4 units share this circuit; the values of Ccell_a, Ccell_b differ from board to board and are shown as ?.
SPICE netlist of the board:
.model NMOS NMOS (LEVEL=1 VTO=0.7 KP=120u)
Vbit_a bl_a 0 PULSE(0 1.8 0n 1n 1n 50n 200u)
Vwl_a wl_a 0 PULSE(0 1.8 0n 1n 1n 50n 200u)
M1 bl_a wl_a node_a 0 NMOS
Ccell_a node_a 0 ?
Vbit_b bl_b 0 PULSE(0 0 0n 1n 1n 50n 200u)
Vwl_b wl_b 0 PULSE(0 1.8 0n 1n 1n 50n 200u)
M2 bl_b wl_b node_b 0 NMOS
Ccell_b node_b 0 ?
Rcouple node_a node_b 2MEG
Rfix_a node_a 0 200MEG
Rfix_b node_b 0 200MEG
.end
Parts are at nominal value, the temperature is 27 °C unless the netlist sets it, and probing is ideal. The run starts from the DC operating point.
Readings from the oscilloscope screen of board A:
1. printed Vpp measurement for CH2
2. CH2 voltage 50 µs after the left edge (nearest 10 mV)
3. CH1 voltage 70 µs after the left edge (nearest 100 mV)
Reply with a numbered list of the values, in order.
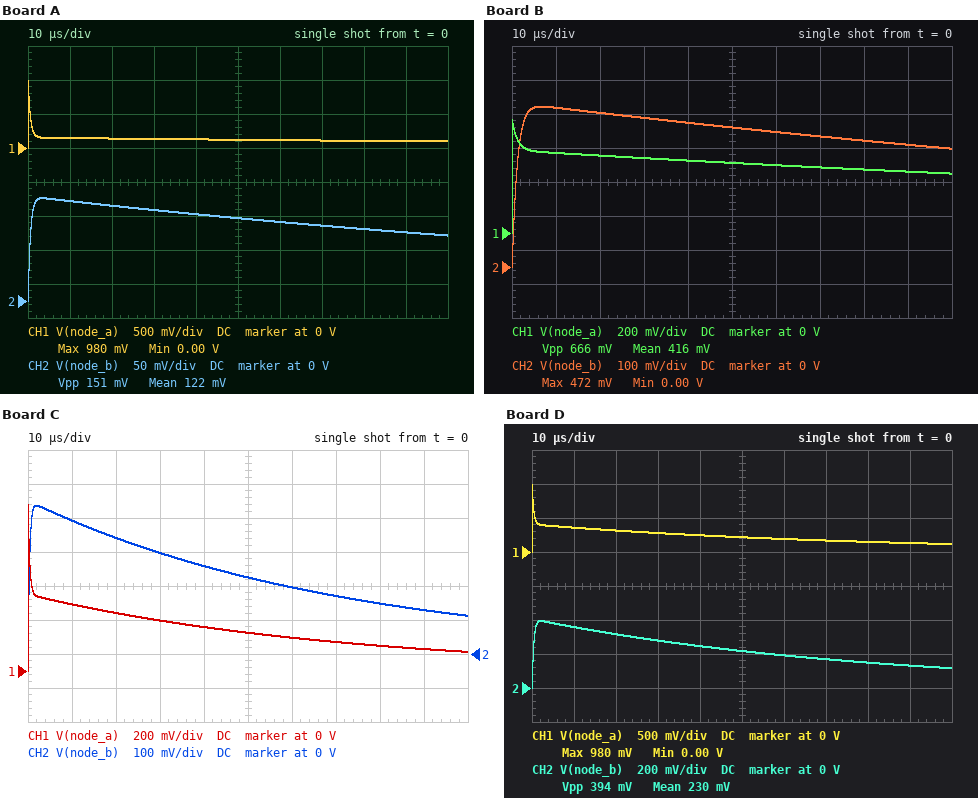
1. 151 mV
2. 120 mV
3. 100 mV
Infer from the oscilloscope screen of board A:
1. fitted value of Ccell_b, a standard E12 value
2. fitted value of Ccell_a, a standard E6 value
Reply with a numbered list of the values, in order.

1. 1.8 pF
2. 330 fF
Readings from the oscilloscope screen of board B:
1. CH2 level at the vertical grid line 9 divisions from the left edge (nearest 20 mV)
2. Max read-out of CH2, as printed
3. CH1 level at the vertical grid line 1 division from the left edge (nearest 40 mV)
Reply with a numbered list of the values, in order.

1. 360 mV
2. 472 mV
3. 480 mV
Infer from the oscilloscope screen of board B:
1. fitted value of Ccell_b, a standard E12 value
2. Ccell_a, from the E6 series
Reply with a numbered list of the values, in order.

1. 820 fF
2. 2.2 pF
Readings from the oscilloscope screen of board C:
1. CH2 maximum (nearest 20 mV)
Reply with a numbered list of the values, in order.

1. 440 mV
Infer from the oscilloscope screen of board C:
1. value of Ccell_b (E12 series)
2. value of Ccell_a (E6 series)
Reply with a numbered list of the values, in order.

1. 390 fF
2. 330 fF
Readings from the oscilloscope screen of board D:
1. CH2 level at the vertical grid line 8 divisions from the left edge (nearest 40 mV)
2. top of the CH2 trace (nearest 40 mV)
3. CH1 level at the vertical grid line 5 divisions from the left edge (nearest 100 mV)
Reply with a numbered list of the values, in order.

1. 160 mV
2. 400 mV
3. 200 mV
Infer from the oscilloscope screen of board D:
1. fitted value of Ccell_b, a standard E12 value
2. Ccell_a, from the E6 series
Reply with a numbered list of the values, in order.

1. 470 fF
2. 330 fF
